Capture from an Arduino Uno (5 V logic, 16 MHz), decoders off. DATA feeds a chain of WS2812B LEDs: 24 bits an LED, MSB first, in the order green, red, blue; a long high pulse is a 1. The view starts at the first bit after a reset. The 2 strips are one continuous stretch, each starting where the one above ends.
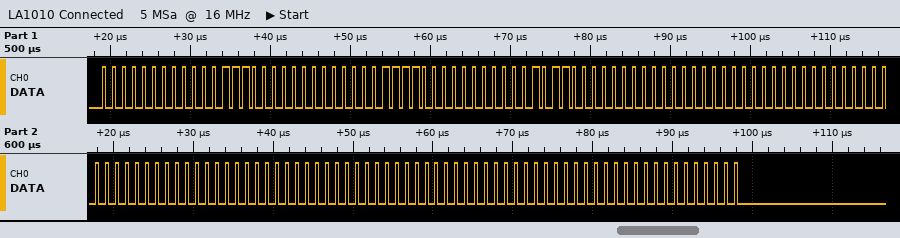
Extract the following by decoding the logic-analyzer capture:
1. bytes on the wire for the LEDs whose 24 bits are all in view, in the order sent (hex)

00 0E 00 0F 00 16 00 00 00 00 00 00 00 00 00 00 00 00
